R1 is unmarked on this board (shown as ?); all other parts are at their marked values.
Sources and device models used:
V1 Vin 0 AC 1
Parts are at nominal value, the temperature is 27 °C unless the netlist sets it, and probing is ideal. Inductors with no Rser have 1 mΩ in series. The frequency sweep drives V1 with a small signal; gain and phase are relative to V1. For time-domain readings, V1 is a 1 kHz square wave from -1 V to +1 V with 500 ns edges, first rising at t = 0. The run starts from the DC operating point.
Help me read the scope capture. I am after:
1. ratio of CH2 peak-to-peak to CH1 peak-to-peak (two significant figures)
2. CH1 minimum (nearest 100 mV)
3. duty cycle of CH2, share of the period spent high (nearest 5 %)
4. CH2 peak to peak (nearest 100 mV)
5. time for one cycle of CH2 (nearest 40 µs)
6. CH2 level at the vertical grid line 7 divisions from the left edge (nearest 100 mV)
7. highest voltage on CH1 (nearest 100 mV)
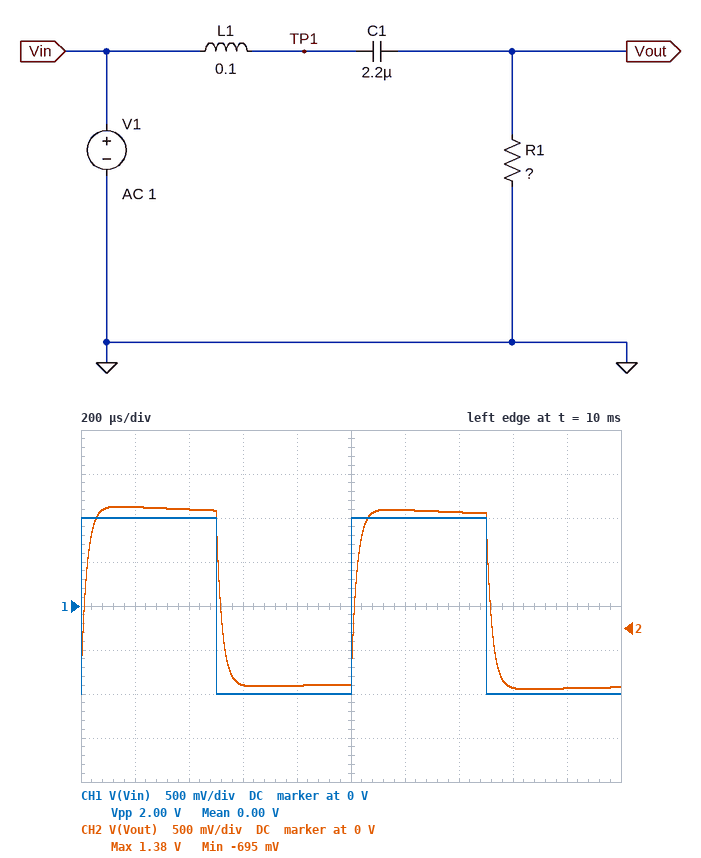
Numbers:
1.0
-1.0 V
50 %
2.1 V
1.00 ms
1.3 V
1.0 V
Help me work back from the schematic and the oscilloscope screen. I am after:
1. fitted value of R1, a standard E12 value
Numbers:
4.7 kΩ
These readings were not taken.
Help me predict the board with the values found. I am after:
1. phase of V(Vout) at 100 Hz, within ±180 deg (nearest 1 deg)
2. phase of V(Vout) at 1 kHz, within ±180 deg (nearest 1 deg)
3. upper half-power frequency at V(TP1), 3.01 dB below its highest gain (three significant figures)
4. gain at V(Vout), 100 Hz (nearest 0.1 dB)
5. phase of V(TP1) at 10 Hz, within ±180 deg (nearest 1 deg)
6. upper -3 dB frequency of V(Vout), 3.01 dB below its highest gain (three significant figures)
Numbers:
8 deg
-7 deg
7.47 kHz
-0.1 dB
0 deg
7.50 kHz
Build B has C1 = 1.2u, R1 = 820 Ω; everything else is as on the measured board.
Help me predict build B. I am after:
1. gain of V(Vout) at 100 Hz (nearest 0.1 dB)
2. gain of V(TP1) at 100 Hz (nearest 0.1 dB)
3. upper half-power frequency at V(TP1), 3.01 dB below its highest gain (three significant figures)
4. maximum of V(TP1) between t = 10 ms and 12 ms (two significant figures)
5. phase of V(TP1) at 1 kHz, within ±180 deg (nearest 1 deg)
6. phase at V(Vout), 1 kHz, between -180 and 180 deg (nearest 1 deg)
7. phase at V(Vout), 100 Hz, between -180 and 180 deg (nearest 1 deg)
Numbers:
-5.3 dB
0.3 dB
1.28 kHz
1.1 V
-40 deg
-31 deg
57 deg
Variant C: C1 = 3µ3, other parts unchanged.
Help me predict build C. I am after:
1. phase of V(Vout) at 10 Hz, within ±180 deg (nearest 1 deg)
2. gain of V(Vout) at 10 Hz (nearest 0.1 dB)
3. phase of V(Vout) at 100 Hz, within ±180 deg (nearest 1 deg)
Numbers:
46 deg
-3.1 dB
5 deg
